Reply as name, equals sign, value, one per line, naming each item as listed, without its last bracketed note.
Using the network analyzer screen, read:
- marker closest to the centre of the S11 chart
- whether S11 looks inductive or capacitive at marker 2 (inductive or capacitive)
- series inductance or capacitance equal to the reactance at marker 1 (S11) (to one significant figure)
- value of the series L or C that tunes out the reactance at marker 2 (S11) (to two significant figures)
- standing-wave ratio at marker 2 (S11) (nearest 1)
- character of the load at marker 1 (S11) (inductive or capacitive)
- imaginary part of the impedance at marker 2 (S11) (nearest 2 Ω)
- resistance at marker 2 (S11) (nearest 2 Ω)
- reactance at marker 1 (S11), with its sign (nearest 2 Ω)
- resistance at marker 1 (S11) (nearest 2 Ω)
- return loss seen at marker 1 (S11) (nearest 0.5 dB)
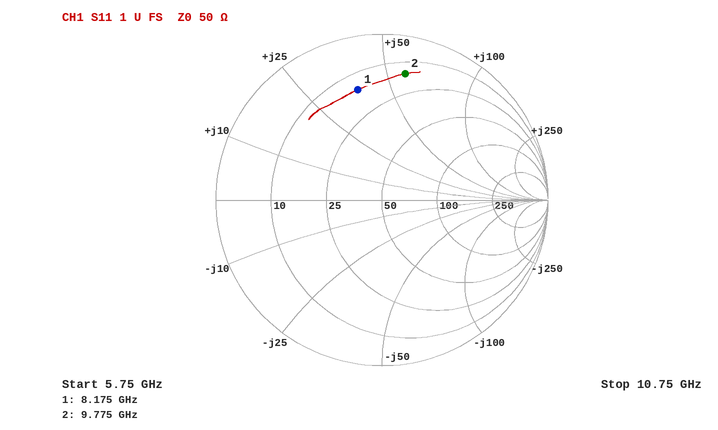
marker closest to the centre of the S11 chart = marker 1
whether S11 looks inductive or capacitive at marker 2 = inductive
series inductance or capacitance equal to the reactance at marker 1 (S11) = 700 pH
value of the series L or C that tunes out the reactance at marker 2 (S11) = 280 fF
standing-wave ratio at marker 2 (S11) = 8
character of the load at marker 1 (S11) = inductive
imaginary part of the impedance at marker 2 (S11) = +58 Ω
resistance at marker 2 (S11) = 16 Ω
reactance at marker 1 (S11), with its sign = +38 Ω
resistance at marker 1 (S11) = 16 Ω
return loss seen at marker 1 (S11) = 3.5 dB
